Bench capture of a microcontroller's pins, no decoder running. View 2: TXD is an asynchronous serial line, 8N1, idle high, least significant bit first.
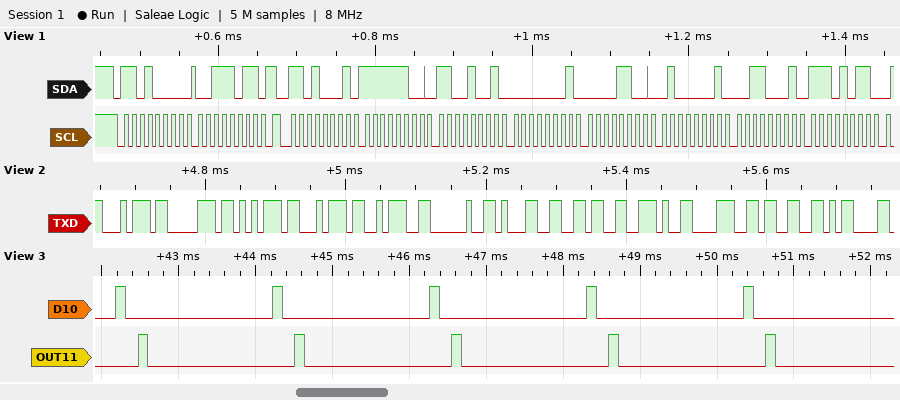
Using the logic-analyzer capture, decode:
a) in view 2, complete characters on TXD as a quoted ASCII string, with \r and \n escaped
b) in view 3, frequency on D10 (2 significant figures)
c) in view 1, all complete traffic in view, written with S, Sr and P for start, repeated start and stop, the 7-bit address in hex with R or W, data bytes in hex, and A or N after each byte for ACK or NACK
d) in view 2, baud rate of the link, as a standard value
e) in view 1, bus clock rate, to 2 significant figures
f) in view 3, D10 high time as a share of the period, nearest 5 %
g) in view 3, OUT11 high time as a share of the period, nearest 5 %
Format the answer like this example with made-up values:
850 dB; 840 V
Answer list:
"tput: 16.83\r"; 490 Hz; S 68W A 3B A Sr 68R A FC A C9 A 01 A 0C A 41 A 31 A EB A; 115200 baud; 100 kHz; 5 %; 5 %
